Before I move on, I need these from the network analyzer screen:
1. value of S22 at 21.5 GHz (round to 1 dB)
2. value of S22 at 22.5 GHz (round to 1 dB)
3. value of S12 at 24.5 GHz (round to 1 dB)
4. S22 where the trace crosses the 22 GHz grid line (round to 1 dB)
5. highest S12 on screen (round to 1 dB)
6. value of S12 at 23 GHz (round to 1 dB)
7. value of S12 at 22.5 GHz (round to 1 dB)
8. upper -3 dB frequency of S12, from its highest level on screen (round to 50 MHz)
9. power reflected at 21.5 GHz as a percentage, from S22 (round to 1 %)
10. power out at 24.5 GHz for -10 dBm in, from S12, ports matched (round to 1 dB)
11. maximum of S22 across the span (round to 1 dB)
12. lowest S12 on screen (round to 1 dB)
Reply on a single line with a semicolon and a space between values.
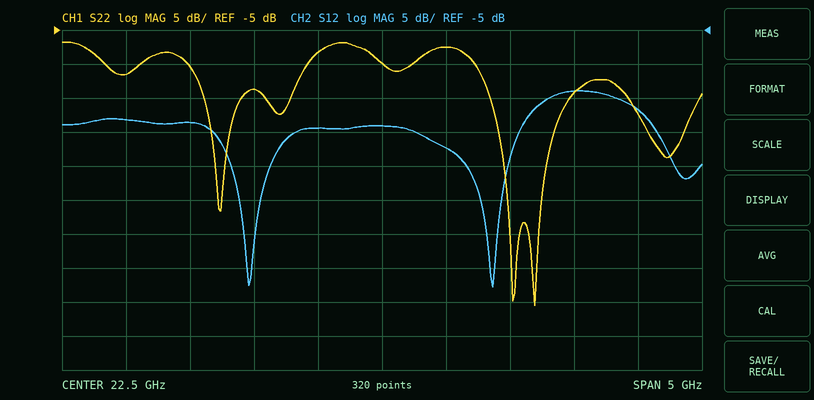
-14 dB; -10 dB; -17 dB; -8 dB; -14 dB; -22 dB; -19 dB; 24.50 GHz; 4 %; -27 dBm; -7 dB; -43 dB
